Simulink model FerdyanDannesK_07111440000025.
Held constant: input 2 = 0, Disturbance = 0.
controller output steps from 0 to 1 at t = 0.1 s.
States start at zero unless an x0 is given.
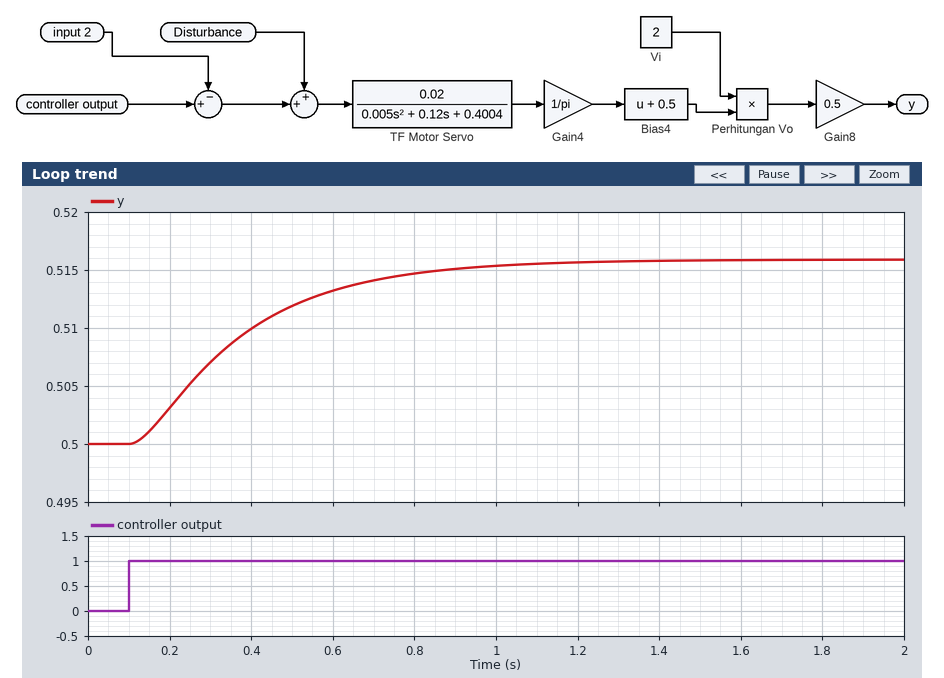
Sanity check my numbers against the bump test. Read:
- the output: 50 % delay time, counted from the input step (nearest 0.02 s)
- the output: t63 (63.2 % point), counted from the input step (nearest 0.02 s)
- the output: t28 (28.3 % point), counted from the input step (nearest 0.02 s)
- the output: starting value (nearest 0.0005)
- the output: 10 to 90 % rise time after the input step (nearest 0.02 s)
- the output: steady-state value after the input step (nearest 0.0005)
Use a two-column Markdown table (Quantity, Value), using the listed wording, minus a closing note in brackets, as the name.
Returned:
| Quantity | Value |
|---|---|
| the output: 50 % delay time, counted from the input step | 0.22 s |
| the output: t63 (63.2 % point), counted from the input step | 0.30 s |
| the output: t28 (28.3 % point), counted from the input step | 0.14 s |
| the output: starting value | 0.5000 |
| the output: 10 to 90 % rise time after the input step | 0.56 s |
| the output: steady-state value after the input step | 0.5160 |
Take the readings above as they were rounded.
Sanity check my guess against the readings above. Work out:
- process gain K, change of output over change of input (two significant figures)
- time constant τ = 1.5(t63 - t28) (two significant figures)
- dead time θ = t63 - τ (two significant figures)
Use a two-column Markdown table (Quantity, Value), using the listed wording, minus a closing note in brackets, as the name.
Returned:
| Quantity | Value |
|---|---|
| process gain K, change of output over change of input | 0.016 |
| time constant τ = 1.5(t63 - t28) | 0.24 s |
| dead time θ = t63 - τ | 0.060 s |
